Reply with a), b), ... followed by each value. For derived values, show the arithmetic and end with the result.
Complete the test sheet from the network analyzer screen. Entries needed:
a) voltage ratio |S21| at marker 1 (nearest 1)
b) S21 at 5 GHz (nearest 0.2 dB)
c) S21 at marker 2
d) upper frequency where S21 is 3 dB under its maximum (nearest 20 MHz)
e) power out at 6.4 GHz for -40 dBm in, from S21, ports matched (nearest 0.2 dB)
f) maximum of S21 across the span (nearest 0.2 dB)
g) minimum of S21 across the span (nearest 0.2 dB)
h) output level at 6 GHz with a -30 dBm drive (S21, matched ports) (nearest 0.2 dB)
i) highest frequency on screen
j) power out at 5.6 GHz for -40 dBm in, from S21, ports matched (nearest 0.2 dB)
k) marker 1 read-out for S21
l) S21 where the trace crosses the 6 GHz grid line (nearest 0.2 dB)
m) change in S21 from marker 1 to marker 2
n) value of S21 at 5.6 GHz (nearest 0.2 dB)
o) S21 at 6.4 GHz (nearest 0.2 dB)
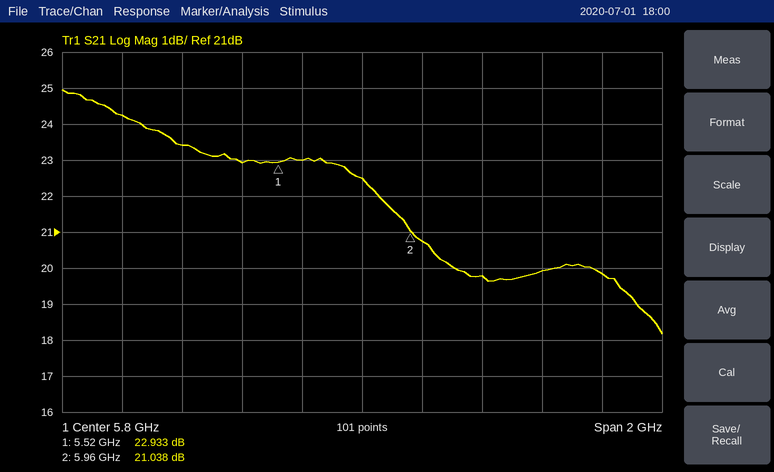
a) 10^(22.933/20) ≈ 14
b) 24.2 dB
c) 21.038 dB
d) 5.86 GHz
e) -40 dBm + (20.0 dB) = -20.0 dBm
f) 25.0 dB
g) 18.2 dB
h) -30 dBm + (20.8 dB) = -9.2 dBm
i) 6.8 GHz
j) -40 dBm + (23.0 dB) = -17.0 dBm
k) 22.933 dB
l) 20.8 dB
m) 21.038 − (22.933) = -1.895 dB
n) 23.0 dB
o) 20.0 dB
